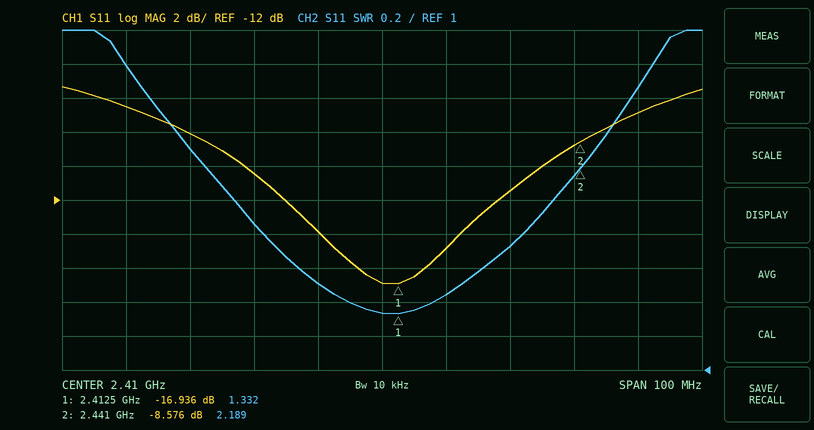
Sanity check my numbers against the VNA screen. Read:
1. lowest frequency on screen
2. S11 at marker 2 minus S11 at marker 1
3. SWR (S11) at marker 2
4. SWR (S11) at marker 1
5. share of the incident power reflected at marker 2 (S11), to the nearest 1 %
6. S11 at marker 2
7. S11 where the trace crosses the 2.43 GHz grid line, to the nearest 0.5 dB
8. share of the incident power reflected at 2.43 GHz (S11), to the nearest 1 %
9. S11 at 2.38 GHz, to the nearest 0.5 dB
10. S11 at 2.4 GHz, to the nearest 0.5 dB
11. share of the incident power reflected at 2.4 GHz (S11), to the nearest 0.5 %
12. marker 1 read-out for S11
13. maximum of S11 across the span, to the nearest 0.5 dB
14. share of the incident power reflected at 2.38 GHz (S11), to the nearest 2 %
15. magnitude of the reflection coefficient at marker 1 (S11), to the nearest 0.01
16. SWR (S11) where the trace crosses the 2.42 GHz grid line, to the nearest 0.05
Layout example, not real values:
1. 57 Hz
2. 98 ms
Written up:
1. 2.36 GHz
2. 8.360 dB
3. 2.189
4. 1.332
5. 14 %
6. -8.576 dB
7. -11.5 dB
8. 7 %
9. -8.0 dB
10. -14.0 dB
11. 4.0 %
12. -16.936 dB
13. -5.5 dB
14. 16 %
15. 0.14
16. 1.45
